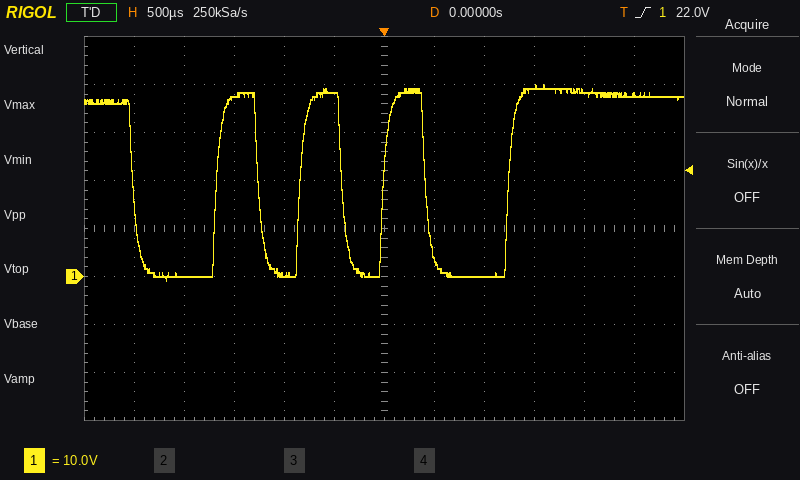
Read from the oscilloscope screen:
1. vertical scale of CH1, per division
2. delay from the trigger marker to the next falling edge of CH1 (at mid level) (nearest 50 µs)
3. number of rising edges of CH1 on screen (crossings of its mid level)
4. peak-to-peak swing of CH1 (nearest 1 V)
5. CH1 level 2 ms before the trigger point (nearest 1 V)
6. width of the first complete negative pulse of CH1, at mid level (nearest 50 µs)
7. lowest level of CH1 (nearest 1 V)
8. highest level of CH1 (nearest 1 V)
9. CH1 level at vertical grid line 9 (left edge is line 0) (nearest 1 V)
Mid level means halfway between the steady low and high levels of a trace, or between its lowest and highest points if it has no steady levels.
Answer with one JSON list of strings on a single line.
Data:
["10 V", "400 µs", "4", "41 V", "0 V", "850 µs", "-1 V", "40 V", "40 V"]
